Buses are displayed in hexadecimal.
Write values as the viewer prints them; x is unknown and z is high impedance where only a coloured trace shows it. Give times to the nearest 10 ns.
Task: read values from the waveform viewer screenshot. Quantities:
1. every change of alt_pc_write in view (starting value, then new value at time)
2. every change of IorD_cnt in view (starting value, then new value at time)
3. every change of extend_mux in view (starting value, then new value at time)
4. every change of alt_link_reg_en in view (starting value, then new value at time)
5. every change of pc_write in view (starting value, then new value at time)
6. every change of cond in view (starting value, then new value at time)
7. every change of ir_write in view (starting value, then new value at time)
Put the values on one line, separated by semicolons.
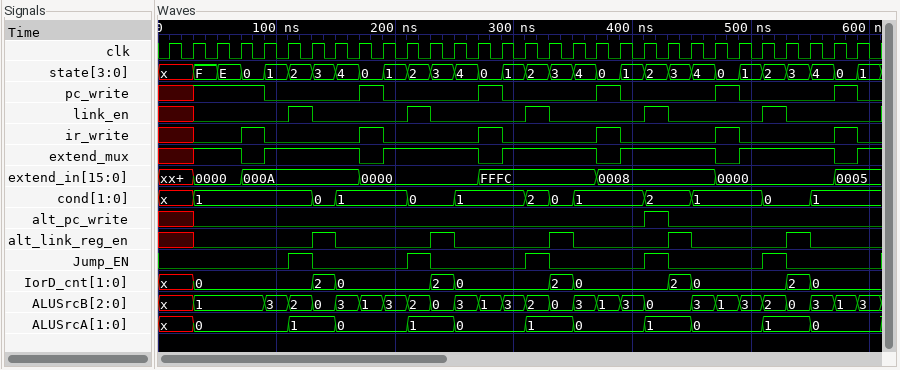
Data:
x, 0 at 30 ns, 1 at 410 ns, 0 at 430 ns; x, 0 at 30 ns, 2 at 130 ns, 0 at 150 ns, 2 at 230 ns, 0 at 250 ns, 2 at 330 ns, 0 at 350 ns, 2 at 430 ns, 0 at 450 ns, 2 at 530 ns, 0 at 550 ns; x, 1 at 30 ns, 0 at 70 ns, 1 at 90 ns, 0 at 170 ns, 1 at 190 ns, 0 at 270 ns, 1 at 290 ns, 0 at 370 ns, 1 at 390 ns, 0 at 470 ns, 1 at 490 ns, 0 at 570 ns, 1 at 590 ns; x, 0 at 30 ns, 1 at 130 ns, 0 at 150 ns, 1 at 230 ns, 0 at 250 ns, 1 at 330 ns, 0 at 350 ns, 1 at 430 ns, 0 at 450 ns, 1 at 530 ns, 0 at 550 ns; x, 1 at 30 ns, 0 at 90 ns, 1 at 170 ns, 0 at 190 ns, 1 at 270 ns, 0 at 290 ns, 1 at 370 ns, 0 at 390 ns, 1 at 470 ns, 0 at 490 ns, 1 at 570 ns, 0 at 590 ns; x, 1 at 30 ns, 0 at 130 ns, 1 at 150 ns, 0 at 210 ns, 1 at 250 ns, 2 at 310 ns, 0 at 330 ns, 1 at 350 ns, 2 at 410 ns, 1 at 450 ns, 0 at 510 ns, 1 at 550 ns; x, 0 at 30 ns, 1 at 70 ns, 0 at 90 ns, 1 at 170 ns, 0 at 190 ns, 1 at 270 ns, 0 at 290 ns, 1 at 370 ns, 0 at 390 ns, 1 at 470 ns, 0 at 490 ns, 1 at 570 ns, 0 at 590 ns
